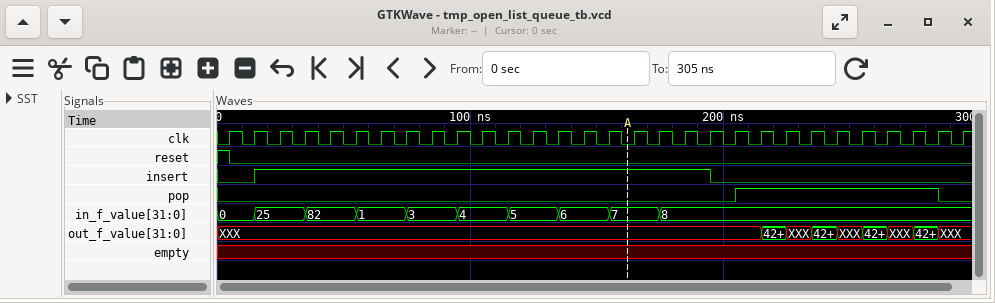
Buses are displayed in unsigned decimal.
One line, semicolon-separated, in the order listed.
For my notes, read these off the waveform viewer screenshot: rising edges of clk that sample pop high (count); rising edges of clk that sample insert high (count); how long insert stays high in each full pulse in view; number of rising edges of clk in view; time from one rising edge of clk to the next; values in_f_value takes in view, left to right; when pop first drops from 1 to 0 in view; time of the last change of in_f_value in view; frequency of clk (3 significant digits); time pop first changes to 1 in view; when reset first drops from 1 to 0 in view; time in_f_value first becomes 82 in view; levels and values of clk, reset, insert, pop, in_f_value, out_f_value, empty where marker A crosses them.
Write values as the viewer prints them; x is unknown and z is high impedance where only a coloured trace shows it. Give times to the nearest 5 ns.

8; 18; 180 ns; 30; 10 ns; 0, 25, 82, 1, 3, 4, 5, 6, 7, 8; 285 ns; 175 ns; 100 MHz; 205 ns; 5 ns; 35 ns; clk=0, reset=0, insert=1, pop=0, in_f_value=7, out_f_value=XXX, empty=x
